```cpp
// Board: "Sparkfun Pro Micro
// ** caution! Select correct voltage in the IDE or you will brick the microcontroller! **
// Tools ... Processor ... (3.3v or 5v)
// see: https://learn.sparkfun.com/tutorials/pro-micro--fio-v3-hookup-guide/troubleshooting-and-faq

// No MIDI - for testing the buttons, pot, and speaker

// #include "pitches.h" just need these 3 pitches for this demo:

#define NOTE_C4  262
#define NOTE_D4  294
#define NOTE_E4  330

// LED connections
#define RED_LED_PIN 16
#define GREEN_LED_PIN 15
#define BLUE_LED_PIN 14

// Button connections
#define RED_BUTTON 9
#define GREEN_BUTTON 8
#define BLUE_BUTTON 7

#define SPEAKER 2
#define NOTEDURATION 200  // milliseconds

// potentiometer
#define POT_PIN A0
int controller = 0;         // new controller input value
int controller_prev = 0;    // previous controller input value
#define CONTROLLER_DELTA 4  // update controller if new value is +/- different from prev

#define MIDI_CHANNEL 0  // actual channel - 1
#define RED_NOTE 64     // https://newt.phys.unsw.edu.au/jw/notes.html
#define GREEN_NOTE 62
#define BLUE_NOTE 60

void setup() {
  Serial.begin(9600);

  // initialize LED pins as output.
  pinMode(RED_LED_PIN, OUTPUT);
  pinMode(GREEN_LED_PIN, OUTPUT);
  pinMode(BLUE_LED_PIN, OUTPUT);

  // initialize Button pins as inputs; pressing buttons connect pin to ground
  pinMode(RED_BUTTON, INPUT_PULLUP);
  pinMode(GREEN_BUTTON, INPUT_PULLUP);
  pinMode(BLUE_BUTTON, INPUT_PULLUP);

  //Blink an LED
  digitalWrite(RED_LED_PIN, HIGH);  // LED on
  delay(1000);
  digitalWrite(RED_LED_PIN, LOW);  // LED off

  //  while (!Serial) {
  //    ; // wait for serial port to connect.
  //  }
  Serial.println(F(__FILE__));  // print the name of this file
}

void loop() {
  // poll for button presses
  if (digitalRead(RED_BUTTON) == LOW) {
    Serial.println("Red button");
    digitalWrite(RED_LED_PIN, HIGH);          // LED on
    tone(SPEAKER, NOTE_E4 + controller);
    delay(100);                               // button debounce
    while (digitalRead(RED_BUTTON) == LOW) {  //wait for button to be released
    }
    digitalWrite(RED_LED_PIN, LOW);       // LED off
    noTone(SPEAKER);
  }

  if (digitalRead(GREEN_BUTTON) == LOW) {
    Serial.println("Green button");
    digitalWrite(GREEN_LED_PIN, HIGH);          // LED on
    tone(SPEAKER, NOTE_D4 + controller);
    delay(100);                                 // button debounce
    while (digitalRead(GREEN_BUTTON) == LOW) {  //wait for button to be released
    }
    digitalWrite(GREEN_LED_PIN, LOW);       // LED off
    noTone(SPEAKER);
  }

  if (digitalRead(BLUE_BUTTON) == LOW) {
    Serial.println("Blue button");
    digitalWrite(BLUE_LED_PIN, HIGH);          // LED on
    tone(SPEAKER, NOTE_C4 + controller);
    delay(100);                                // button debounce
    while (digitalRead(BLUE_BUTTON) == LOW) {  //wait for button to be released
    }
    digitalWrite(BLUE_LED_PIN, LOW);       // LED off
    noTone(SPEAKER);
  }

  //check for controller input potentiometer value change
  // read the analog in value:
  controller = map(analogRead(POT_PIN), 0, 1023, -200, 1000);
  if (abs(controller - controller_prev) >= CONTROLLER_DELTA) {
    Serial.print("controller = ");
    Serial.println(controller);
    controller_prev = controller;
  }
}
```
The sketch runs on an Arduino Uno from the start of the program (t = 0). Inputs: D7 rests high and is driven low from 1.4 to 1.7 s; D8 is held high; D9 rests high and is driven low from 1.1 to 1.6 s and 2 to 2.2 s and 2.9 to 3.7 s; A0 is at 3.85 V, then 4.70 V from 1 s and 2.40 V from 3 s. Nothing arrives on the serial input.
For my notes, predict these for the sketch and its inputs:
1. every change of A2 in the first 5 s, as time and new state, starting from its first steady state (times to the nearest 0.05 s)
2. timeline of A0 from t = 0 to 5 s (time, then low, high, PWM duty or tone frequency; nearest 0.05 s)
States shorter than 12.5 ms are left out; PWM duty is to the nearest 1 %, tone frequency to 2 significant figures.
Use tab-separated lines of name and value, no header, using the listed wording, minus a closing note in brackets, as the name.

every change of A2 in the first 5 s, as time and new state, starting from its first steady state	0 s high; 1 s low; 1.1 s high; 1.6 s low; 2 s high; 2.2 s low; 2.9 s high; 3.7 s low
timeline of A0 from t = 0 to 5 s	0 s low; 1.6 s high; 1.7 s low
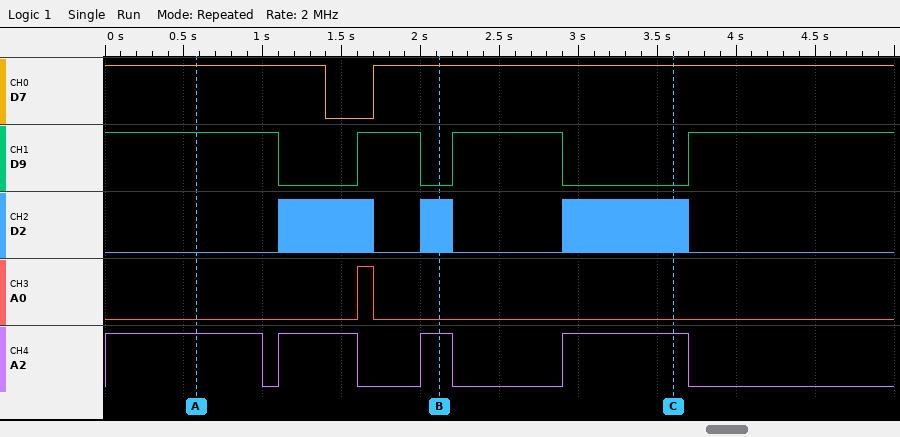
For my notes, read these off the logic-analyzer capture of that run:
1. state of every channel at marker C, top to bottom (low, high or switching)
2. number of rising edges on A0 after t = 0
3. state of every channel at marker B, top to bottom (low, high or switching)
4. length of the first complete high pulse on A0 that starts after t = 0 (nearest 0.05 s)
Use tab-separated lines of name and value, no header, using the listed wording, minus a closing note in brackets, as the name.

state of every channel at marker C, top to bottom	D7 high, D9 low, D2 switching, A0 low, A2 high
number of rising edges on A0 after t = 0	1
state of every channel at marker B, top to bottom	D7 high, D9 low, D2 switching, A0 low, A2 high
length of the first complete high pulse on A0 that starts after t = 0	0.10 s
